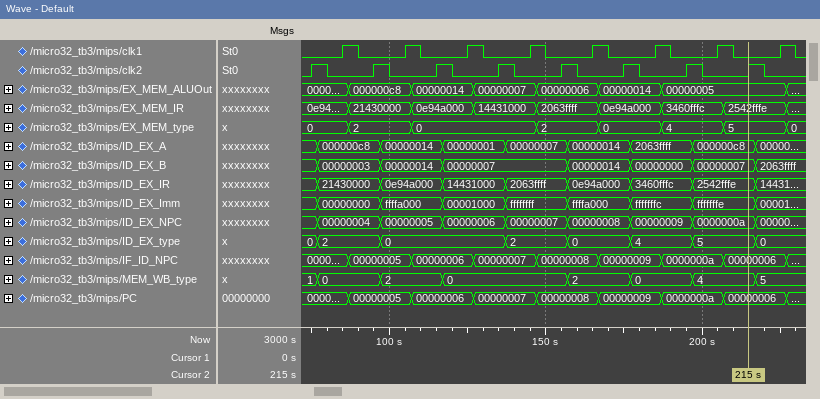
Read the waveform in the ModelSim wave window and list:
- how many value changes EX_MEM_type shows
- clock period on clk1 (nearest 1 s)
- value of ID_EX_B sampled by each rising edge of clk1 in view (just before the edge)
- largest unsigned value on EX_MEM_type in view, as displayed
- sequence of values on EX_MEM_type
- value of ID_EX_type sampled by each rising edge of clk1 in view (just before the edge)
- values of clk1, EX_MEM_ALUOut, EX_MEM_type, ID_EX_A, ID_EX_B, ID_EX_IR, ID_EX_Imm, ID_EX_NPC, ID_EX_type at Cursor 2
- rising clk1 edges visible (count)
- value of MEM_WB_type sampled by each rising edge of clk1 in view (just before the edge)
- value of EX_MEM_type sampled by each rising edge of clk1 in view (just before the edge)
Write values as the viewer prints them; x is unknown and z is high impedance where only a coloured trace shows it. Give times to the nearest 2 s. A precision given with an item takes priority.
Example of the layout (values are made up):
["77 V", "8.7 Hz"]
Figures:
["7", "20 s", "00000003, 00000014, 00000007, 00000007, 00000014, 00000000, 00000007, 2063ffff", "5", "0, 2, 0, 2, 0, 4, 5, 0", "2, 0, 0, 2, 0, 4, 5, 0", "clk1=0, EX_MEM_ALUOut=00000005, EX_MEM_type=5, ID_EX_A=000000c8, ID_EX_B=00000007, ID_EX_IR=2542fffe, ID_EX_Imm=fffffffe, ID_EX_NPC=0000000a, ID_EX_type=5", "8", "0, 2, 0, 0, 2, 0, 4, 5", "0, 2, 0, 0, 2, 0, 4, 5"]
